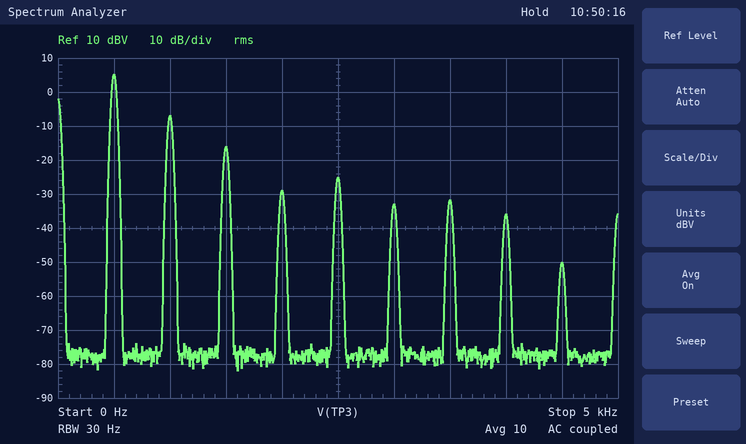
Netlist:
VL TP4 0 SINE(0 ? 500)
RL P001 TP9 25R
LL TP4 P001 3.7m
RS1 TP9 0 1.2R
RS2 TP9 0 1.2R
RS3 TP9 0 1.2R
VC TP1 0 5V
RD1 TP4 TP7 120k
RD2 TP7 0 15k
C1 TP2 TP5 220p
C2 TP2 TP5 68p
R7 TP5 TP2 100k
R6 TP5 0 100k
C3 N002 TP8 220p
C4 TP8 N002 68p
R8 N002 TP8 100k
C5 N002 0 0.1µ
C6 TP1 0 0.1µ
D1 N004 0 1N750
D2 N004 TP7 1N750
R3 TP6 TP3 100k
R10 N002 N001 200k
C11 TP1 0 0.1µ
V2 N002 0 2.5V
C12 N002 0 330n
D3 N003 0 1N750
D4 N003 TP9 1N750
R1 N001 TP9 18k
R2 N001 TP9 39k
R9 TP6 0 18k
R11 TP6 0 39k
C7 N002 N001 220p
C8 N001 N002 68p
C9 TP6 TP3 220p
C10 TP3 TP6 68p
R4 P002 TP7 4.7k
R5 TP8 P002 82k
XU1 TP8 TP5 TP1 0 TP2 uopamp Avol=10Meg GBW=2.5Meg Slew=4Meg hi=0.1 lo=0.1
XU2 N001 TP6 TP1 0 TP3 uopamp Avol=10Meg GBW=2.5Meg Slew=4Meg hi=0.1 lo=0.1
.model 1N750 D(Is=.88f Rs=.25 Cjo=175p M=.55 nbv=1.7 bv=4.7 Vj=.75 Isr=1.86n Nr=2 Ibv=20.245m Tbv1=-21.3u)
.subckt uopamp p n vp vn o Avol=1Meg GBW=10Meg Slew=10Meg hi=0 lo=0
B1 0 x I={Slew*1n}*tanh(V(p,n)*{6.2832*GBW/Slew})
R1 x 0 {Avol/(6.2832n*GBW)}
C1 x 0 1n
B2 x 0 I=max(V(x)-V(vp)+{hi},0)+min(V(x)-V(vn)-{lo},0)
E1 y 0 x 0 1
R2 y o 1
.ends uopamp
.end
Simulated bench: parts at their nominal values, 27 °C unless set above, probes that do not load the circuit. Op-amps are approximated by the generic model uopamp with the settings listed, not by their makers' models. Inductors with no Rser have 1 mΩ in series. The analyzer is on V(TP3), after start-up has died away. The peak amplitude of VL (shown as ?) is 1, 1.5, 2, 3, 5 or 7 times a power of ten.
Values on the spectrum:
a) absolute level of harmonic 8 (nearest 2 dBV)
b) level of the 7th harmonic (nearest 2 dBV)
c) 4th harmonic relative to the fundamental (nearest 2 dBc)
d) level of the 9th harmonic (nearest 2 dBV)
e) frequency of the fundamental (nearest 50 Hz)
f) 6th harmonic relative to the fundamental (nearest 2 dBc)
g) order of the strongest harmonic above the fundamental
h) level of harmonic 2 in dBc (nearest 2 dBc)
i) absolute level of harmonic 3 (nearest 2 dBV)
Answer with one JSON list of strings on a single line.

["-36 dBV", "-32 dBV", "-34 dBc", "-50 dBV", "500 Hz", "-38 dBc", "2", "-12 dBc", "-16 dBV"]
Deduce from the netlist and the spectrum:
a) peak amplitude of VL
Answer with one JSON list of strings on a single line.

["30 V"]
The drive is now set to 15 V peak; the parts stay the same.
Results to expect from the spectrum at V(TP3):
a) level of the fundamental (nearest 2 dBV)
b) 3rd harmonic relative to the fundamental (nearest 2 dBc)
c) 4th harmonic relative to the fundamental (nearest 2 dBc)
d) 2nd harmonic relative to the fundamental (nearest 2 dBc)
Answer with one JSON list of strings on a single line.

["2 dBV", "-24 dBc", "-30 dBc", "-20 dBc"]
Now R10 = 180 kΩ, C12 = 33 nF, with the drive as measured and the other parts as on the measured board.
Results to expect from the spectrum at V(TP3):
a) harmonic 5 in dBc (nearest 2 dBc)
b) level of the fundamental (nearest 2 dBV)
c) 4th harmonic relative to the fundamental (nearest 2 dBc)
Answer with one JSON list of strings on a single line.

["-32 dBc", "6 dBV", "-36 dBc"]
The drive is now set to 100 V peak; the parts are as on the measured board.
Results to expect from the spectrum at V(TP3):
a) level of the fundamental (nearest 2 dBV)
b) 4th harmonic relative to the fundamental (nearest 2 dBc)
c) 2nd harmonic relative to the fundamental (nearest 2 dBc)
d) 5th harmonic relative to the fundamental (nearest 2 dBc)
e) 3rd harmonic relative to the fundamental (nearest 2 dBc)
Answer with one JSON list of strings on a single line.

["6 dBV", "-22 dBc", "-20 dBc", "-16 dBc", "-10 dBc"]
